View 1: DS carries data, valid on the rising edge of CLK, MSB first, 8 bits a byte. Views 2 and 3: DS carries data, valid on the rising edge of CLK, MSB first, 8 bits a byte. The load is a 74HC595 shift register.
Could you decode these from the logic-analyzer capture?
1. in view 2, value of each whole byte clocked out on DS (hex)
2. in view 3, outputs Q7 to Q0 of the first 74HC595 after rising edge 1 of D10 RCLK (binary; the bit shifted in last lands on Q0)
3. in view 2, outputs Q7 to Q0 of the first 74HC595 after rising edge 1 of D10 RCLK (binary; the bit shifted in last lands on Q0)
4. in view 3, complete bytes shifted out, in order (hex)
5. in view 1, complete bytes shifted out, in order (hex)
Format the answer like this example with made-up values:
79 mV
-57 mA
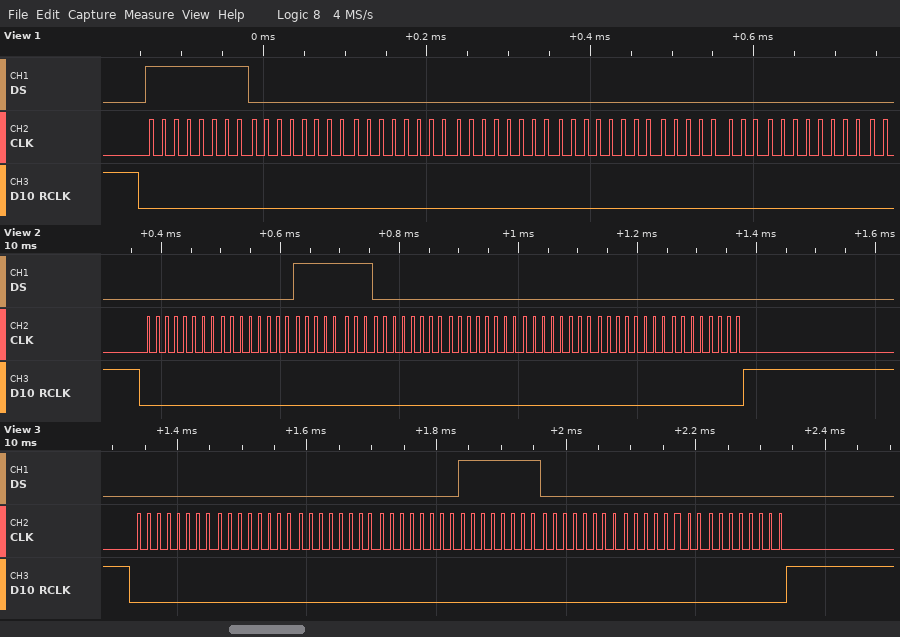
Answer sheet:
00 00 FF 00 00 00 00 00
00000000
00000000
0x00 0x00 0x00 0x00 0xFF 0x00 0x00 0x00
0xFF 0x00 0x00 0x00 0x00 0x00 0x00
